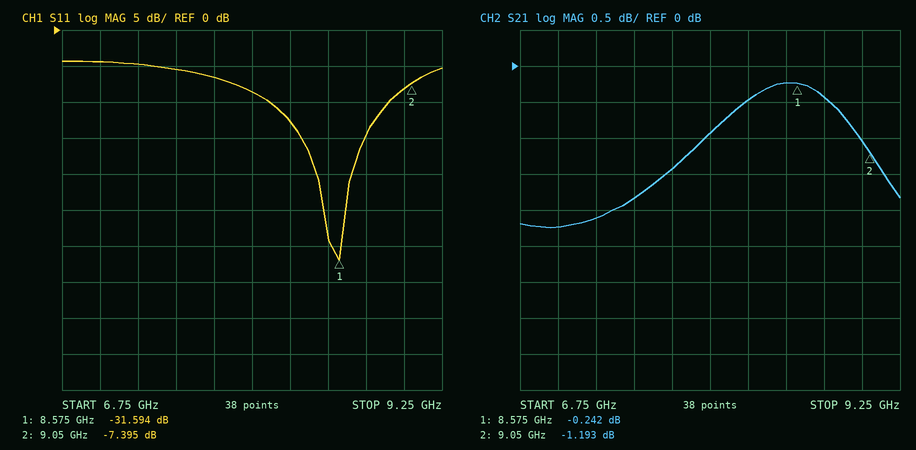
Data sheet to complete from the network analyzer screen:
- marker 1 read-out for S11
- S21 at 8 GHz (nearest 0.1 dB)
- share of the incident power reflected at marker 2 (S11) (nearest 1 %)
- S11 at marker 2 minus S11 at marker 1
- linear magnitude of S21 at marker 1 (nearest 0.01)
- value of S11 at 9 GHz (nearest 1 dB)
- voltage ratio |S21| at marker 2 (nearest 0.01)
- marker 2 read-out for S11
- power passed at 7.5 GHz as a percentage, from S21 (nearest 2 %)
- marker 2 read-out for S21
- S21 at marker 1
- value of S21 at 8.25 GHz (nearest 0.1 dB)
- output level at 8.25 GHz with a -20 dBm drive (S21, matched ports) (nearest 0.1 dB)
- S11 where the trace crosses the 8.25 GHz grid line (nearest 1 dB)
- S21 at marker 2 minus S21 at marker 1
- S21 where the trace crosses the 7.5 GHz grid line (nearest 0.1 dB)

-31.594 dB
-0.9 dB
18 %
24.199 dB
0.97
-8 dB
0.87
-7.395 dB
66 %
-1.193 dB
-0.242 dB
-0.5 dB
-20.5 dBm
-13 dB
-0.951 dB
-1.8 dB
